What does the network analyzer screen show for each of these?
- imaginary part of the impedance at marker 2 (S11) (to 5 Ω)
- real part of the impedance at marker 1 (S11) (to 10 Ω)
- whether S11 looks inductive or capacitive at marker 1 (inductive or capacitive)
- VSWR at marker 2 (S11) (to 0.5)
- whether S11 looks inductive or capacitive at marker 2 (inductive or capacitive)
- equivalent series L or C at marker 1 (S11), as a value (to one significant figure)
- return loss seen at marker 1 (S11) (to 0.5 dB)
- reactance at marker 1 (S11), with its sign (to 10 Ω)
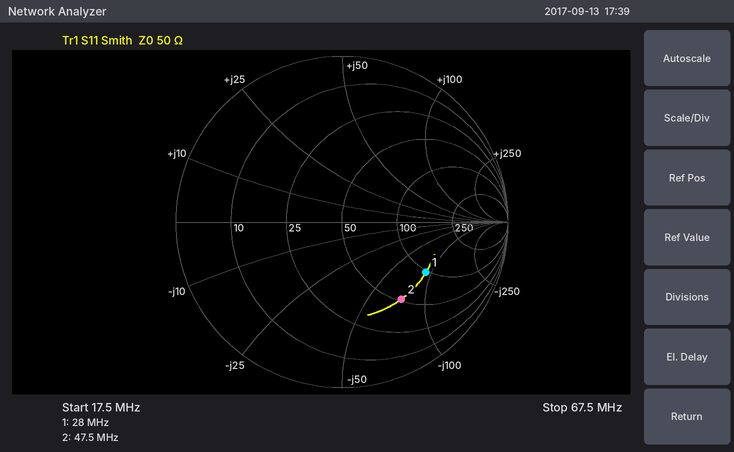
-75 Ω
100 Ω
capacitive
4.0
capacitive
60 pF
4.5 dB
-90 Ω
